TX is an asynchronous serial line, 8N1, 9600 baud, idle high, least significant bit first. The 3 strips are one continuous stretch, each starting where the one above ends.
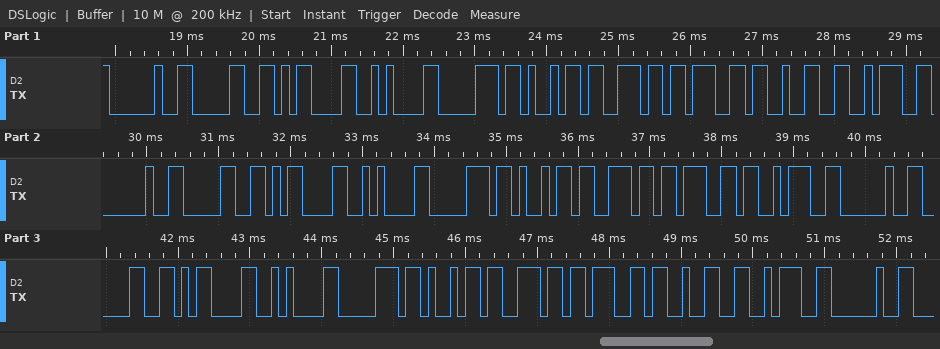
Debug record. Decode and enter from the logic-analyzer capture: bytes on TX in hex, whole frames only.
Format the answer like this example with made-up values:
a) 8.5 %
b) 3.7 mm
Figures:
a) 20 30 0D 0A 70 69 6E 67 32 3A 20 30 0D 0A 70 69 6E 67 3A 20 30 0D 0A 70 69 6E 67 32 3A 20
